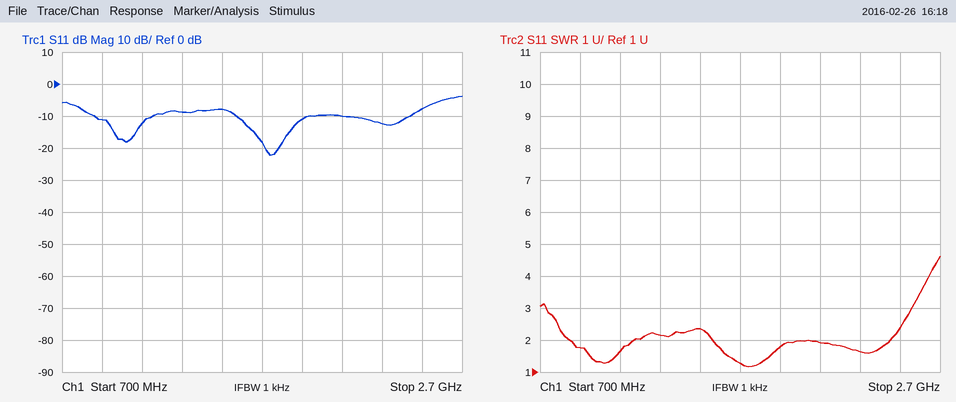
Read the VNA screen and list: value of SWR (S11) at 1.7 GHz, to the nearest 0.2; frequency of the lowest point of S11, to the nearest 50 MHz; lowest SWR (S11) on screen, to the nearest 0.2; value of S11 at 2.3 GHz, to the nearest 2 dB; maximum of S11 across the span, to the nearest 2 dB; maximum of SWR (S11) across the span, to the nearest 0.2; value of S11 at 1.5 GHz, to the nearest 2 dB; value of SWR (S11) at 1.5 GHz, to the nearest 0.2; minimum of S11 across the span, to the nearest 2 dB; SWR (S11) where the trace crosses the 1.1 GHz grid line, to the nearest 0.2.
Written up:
1.2
1.75 GHz
1.2
-12 dB
-4 dB
4.6
-8 dB
2.4
-22 dB
1.6
